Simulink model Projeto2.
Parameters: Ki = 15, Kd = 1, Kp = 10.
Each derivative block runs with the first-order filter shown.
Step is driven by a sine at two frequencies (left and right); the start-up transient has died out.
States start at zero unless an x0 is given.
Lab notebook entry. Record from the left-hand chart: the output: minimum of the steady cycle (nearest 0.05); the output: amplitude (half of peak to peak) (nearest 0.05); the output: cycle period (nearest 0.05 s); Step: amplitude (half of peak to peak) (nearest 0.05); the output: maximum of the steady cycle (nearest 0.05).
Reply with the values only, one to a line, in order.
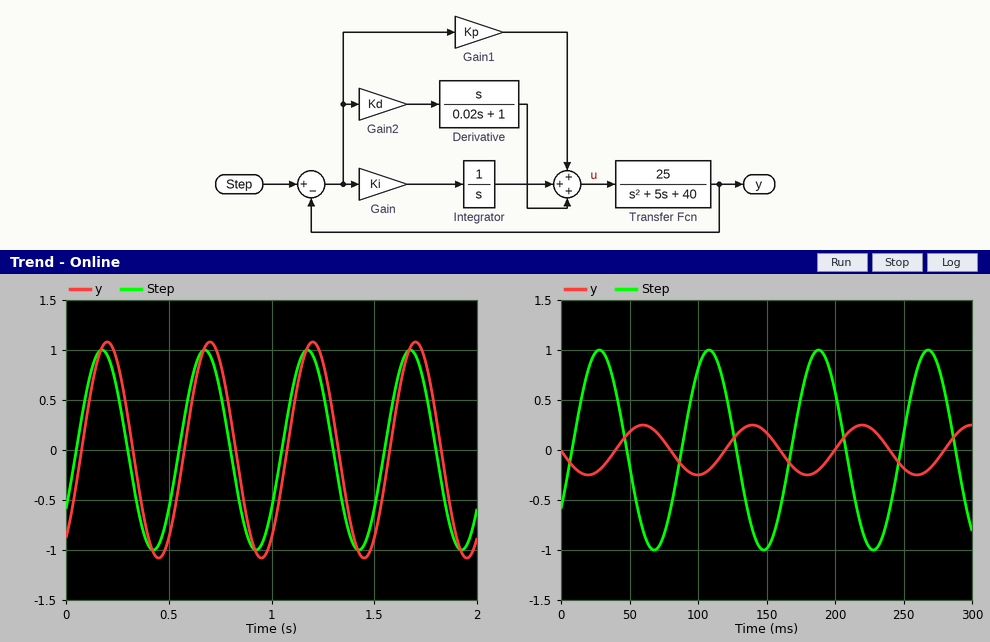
-1.10
1.10
0.50 s
1.00
1.10
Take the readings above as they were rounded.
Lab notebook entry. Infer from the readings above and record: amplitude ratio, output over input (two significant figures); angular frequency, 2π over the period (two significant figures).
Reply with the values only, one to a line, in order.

1.1
13 rad/s
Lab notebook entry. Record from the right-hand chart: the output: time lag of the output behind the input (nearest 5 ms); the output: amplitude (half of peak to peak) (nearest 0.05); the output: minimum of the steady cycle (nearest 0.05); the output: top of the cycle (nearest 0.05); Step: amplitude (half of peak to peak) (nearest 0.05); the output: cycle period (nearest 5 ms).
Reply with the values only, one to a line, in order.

30 ms
0.25
-0.25
0.25
1.00
80 ms
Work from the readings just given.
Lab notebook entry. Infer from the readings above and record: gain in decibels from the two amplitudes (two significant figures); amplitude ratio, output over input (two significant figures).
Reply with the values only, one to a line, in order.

-12 dB
0.25
